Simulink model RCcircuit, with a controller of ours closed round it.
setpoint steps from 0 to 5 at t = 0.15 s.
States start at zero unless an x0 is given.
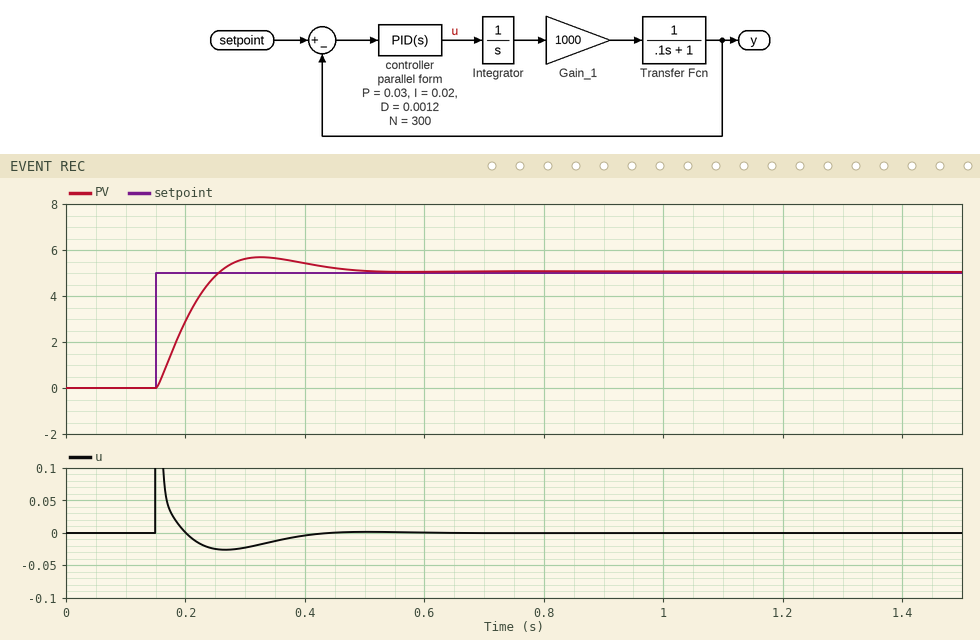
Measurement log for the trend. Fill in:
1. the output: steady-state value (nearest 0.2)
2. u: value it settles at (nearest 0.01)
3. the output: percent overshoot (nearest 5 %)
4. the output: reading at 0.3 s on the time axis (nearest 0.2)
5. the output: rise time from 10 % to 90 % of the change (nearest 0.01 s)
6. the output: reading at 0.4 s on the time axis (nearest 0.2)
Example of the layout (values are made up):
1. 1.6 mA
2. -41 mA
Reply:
1. 5.0
2. 0.00
3. 15 %
4. 5.6
5. 0.08 s
6. 5.4
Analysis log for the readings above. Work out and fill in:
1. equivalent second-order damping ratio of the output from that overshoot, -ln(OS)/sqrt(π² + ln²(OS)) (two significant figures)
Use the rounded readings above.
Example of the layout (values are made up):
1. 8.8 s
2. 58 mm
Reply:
1. 0.52
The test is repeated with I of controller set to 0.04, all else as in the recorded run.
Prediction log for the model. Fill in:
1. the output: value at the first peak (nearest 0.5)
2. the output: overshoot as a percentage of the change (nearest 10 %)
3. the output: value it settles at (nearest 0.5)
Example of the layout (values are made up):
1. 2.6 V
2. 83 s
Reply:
1. 6.0
2. 20 %
3. 5.0
